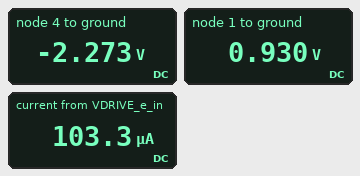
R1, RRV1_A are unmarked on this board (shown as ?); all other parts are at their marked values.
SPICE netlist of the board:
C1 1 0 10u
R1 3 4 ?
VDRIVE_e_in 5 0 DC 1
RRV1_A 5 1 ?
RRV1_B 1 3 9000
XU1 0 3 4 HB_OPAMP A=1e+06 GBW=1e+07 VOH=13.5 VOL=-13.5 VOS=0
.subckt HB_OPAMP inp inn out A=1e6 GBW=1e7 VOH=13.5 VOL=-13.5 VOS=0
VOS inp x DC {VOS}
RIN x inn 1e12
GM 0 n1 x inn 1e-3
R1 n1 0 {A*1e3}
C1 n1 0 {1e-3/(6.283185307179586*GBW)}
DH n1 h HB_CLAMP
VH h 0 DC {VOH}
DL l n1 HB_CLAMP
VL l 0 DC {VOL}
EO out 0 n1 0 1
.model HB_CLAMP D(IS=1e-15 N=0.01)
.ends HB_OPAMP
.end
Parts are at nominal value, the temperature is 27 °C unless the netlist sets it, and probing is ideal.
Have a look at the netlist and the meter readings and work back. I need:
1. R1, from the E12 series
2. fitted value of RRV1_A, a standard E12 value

22 kΩ
680 Ω
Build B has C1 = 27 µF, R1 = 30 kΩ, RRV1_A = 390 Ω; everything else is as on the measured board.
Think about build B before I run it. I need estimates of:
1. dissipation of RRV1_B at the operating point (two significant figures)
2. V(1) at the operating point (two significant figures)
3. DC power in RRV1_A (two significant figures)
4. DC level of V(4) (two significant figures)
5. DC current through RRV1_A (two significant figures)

100 µW
960 mV
4.4 µW
-3.2 V
110 µA
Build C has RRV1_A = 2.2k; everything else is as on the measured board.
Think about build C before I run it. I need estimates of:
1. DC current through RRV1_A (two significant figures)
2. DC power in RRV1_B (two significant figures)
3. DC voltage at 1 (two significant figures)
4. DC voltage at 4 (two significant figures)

89 µA
72 µW
800 mV
-2.0 V
